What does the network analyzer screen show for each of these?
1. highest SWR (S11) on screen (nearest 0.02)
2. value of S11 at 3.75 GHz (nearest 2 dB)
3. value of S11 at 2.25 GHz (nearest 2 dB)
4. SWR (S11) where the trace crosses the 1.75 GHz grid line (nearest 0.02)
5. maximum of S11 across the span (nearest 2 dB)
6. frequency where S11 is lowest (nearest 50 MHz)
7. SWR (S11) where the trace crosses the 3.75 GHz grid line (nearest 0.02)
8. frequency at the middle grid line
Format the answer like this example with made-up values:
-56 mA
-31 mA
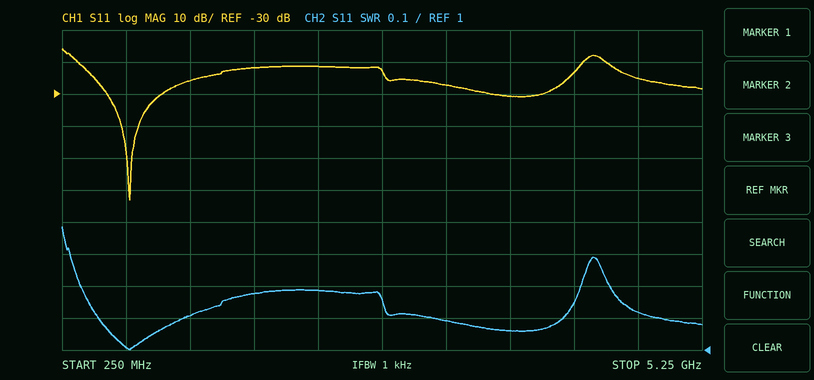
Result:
1.38
-30 dB
-22 dB
1.18
-16 dB
800 MHz
1.06
2.75 GHz
